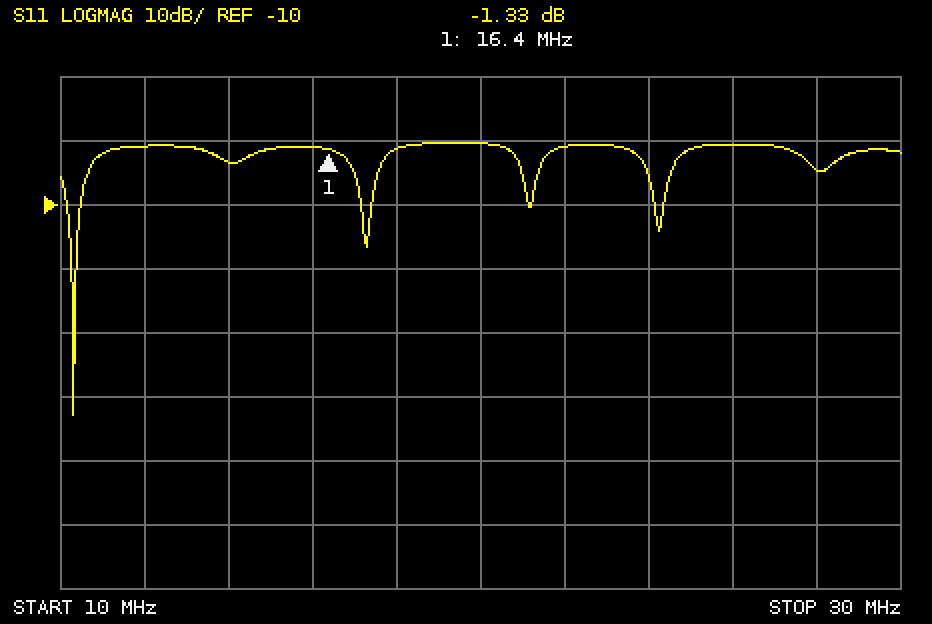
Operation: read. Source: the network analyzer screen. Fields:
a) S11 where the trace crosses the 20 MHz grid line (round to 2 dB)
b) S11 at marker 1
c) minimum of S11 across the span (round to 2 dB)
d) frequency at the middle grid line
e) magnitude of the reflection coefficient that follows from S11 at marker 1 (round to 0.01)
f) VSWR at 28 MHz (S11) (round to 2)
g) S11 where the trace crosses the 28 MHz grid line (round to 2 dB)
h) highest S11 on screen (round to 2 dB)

0 dB
-1.33 dB
-42 dB
20 MHz
0.86
4
-4 dB
0 dB
